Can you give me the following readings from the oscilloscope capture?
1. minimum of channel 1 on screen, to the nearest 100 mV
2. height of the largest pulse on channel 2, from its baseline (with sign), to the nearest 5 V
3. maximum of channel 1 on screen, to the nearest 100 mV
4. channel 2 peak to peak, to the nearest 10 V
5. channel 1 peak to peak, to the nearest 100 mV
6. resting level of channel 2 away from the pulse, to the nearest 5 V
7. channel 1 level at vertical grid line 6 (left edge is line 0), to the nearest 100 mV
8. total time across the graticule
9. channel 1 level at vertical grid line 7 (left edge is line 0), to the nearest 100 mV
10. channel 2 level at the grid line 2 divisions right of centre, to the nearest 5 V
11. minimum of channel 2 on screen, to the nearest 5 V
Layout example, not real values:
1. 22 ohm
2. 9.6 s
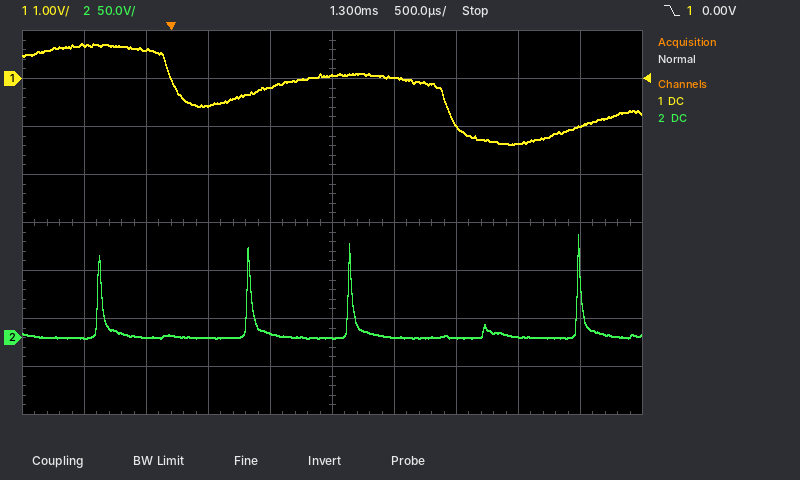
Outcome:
1. -1.4 V
2. +105 V
3. 700 mV
4. 110 V
5. 2.1 V
6. 0 V
7. 0.0 V
8. 5 ms
9. -1.0 V
10. 0 V
11. 0 V
